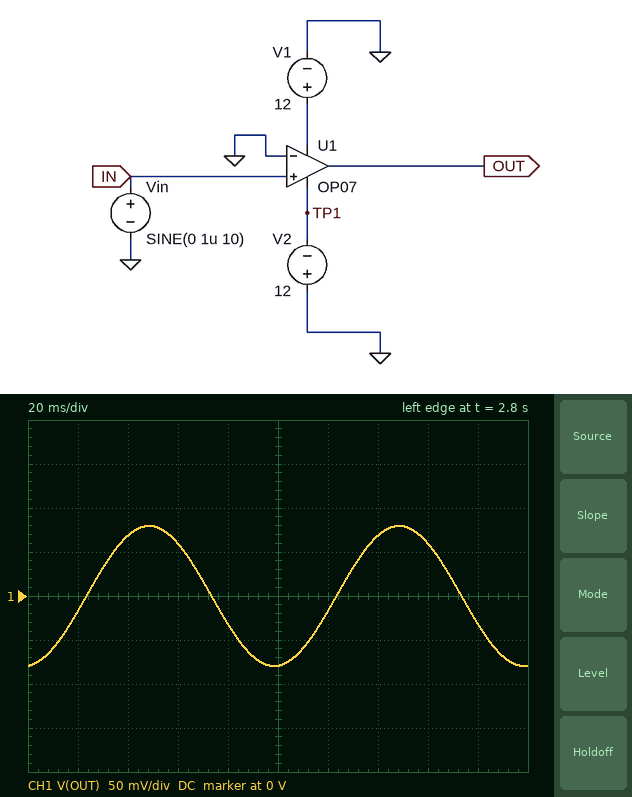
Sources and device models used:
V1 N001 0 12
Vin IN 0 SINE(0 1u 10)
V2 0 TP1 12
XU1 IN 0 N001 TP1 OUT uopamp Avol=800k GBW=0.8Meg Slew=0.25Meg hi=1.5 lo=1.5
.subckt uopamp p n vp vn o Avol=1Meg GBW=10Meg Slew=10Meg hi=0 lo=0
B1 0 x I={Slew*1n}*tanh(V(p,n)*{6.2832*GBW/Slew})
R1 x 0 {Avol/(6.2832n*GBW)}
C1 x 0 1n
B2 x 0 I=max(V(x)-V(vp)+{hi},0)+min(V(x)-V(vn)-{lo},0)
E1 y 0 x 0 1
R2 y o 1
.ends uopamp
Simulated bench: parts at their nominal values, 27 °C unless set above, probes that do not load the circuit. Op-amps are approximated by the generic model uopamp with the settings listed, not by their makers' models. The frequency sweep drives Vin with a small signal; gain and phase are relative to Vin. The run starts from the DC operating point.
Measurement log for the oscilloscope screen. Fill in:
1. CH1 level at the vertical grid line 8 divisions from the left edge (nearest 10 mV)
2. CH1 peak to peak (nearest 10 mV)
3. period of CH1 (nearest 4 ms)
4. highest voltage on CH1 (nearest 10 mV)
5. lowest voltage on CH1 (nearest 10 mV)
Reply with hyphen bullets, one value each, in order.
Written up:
- 60 mV
- 160 mV
- 100 ms
- 80 mV
- -80 mV
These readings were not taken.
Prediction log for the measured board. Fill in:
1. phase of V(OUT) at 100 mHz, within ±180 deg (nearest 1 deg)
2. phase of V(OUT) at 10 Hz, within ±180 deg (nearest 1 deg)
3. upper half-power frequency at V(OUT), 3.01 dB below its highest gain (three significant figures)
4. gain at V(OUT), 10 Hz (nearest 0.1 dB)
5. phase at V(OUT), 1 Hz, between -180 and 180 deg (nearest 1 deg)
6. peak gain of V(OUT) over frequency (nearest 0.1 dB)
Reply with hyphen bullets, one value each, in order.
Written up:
- -6 deg
- -84 deg
- 1.00 Hz
- 98.0 dB
- -45 deg
- 118.1 dB
